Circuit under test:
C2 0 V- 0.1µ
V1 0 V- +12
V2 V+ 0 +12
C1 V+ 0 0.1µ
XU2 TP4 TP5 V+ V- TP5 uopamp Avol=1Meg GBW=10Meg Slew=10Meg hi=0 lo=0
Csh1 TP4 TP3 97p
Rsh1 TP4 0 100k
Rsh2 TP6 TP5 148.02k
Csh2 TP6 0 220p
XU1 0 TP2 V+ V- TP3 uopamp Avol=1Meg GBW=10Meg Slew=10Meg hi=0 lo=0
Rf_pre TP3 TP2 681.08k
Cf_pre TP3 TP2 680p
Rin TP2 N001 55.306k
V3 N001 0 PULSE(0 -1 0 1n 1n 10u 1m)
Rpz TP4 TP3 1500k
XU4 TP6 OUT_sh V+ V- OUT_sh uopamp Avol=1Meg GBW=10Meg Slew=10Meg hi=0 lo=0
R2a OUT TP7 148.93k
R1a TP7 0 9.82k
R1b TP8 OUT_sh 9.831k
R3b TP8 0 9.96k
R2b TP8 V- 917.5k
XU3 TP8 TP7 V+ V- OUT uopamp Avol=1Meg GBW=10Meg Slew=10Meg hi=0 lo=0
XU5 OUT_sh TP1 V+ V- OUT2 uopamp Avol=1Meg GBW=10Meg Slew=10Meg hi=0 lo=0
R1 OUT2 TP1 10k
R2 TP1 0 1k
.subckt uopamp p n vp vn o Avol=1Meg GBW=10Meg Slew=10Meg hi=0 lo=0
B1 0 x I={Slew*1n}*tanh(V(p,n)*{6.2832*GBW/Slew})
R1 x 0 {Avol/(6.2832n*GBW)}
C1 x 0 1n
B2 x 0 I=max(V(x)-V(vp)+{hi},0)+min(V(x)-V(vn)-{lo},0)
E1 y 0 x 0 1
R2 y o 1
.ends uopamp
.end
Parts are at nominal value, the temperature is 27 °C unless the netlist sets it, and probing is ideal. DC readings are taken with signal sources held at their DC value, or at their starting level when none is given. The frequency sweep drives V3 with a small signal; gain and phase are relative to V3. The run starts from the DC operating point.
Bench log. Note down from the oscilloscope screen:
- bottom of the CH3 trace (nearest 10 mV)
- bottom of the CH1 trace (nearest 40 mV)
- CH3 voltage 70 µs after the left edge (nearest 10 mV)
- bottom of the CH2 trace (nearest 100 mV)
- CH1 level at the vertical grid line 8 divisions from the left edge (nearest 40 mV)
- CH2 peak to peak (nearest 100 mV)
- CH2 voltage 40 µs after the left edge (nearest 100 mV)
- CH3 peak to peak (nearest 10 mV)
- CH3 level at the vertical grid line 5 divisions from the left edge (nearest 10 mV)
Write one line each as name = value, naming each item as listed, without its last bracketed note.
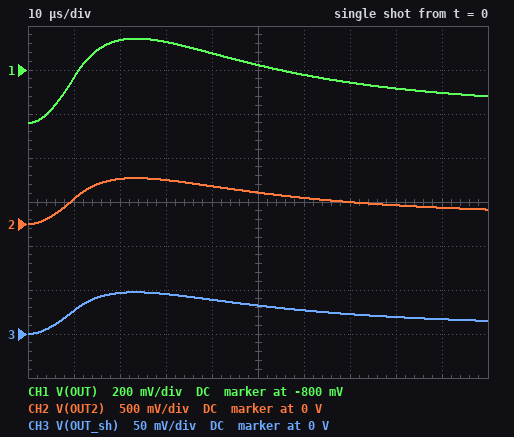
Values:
bottom of the CH3 trace = 0 V
bottom of the CH1 trace = -1.04 V
CH3 voltage 70 µs after the left edge = 20 mV
bottom of the CH2 trace = 0 V
CH1 level at the vertical grid line 8 divisions from the left edge = -880 mV
CH2 peak to peak = 500 mV
CH2 voltage 40 µs after the left edge = 400 mV
CH3 peak to peak = 50 mV
CH3 level at the vertical grid line 5 divisions from the left edge = 30 mV
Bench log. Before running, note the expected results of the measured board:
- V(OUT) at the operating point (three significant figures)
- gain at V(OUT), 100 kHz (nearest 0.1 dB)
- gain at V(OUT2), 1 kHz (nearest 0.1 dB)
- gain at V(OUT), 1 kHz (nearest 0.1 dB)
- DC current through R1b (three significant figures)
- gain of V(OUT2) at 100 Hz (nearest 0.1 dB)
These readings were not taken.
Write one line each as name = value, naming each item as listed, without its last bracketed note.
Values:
V(OUT) at the operating point = -1.04 V
gain at V(OUT), 100 kHz = -35.8 dB
gain at V(OUT2), 1 kHz = 11.2 dB
gain at V(OUT), 1 kHz = 8.6 dB
DC current through R1b = 6.55 µA
gain of V(OUT2) at 100 Hz = 18.2 dB
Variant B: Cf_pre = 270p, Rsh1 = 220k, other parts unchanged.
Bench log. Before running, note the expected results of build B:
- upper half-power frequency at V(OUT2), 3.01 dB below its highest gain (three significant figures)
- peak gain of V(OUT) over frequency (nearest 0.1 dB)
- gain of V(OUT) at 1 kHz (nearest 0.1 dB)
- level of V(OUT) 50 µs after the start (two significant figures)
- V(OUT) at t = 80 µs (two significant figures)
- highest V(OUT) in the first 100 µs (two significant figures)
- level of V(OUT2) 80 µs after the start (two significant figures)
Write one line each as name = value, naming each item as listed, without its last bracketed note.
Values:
upper half-power frequency at V(OUT2), 3.01 dB below its highest gain = 2.39 kHz
peak gain of V(OUT) over frequency = 22.1 dB
gain of V(OUT) at 1 kHz = 20.8 dB
level of V(OUT) 50 µs after the start = 200 mV
V(OUT) at t = 80 µs = -350 mV
highest V(OUT) in the first 100 µs = 450 mV
level of V(OUT2) 80 µs after the start = 940 mV
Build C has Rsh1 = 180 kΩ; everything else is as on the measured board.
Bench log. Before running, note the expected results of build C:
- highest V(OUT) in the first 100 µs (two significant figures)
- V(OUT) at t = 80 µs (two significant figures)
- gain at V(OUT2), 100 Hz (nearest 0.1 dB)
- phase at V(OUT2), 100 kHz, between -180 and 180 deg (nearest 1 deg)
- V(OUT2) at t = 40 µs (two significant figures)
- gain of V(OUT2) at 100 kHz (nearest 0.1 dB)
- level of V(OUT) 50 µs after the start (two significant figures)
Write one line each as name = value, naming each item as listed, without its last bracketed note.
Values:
highest V(OUT) in the first 100 µs = -480 mV
V(OUT) at t = 80 µs = -740 mV
gain at V(OUT2), 100 Hz = 22.9 dB
phase at V(OUT2), 100 kHz, between -180 and 180 deg = 0 deg
V(OUT2) at t = 40 µs = 720 mV
gain of V(OUT2) at 100 kHz = -33.0 dB
level of V(OUT) 50 µs after the start = -570 mV
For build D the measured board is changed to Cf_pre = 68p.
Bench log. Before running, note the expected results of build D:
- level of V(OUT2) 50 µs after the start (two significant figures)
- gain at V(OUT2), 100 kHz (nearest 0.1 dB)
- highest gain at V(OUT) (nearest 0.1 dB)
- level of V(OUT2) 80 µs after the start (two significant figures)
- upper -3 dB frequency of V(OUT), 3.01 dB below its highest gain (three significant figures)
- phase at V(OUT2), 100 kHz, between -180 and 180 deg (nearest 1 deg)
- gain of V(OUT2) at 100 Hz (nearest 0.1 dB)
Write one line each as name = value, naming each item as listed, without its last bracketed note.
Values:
level of V(OUT2) 50 µs after the start = 1.2 V
gain at V(OUT2), 100 kHz = -13.1 dB
highest gain at V(OUT) = 21.3 dB
level of V(OUT2) 80 µs after the start = -280 mV
upper -3 dB frequency of V(OUT), 3.01 dB below its highest gain = 8.42 kHz
phase at V(OUT2), 100 kHz, between -180 and 180 deg = 6 deg
gain of V(OUT2) at 100 Hz = 18.6 dB
